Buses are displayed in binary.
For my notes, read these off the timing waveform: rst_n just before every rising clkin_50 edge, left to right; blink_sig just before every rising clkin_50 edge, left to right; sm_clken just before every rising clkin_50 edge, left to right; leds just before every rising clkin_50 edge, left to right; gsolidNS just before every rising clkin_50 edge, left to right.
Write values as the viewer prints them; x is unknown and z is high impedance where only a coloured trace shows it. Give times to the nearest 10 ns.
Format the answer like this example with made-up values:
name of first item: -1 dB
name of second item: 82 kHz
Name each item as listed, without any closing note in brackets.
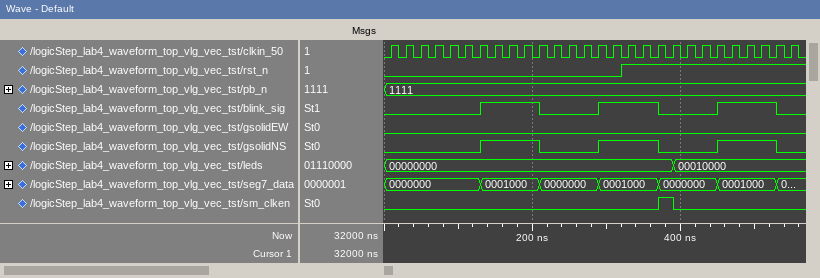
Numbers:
rst_n just before every rising clkin_50 edge, left to right: 0 0 0 0 0 0 0 0 0 0 0 0 0 0 0 0 1 1 1 1 1 1 1 1 1 1 1 1
blink_sig just before every rising clkin_50 edge, left to right: 0 0 0 0 0 0 0 1 1 1 1 0 0 0 0 1 1 1 1 0 0 0 0 1 1 1 1 0
sm_clken just before every rising clkin_50 edge, left to right: 0 0 0 0 0 0 0 0 0 0 0 0 0 0 0 0 0 0 0 1 0 0 0 0 0 0 0 0
leds just before every rising clkin_50 edge, left to right: 00000000, 00000000, 00000000, 00000000, 00000000, 00000000, 00000000, 00000000, 00000000, 00000000, 00000000, 00000000, 00000000, 00000000, 00000000, 00000000, 00000000, 00000000, 00000000, 00000000, 00010000, 00010000, 00010000, 00010000, 00010000, 00010000, 00010000, 00010000
gsolidNS just before every rising clkin_50 edge, left to right: 0 0 0 0 0 0 0 1 1 1 1 0 0 0 0 1 1 1 1 0 0 0 0 1 1 1 1 0
